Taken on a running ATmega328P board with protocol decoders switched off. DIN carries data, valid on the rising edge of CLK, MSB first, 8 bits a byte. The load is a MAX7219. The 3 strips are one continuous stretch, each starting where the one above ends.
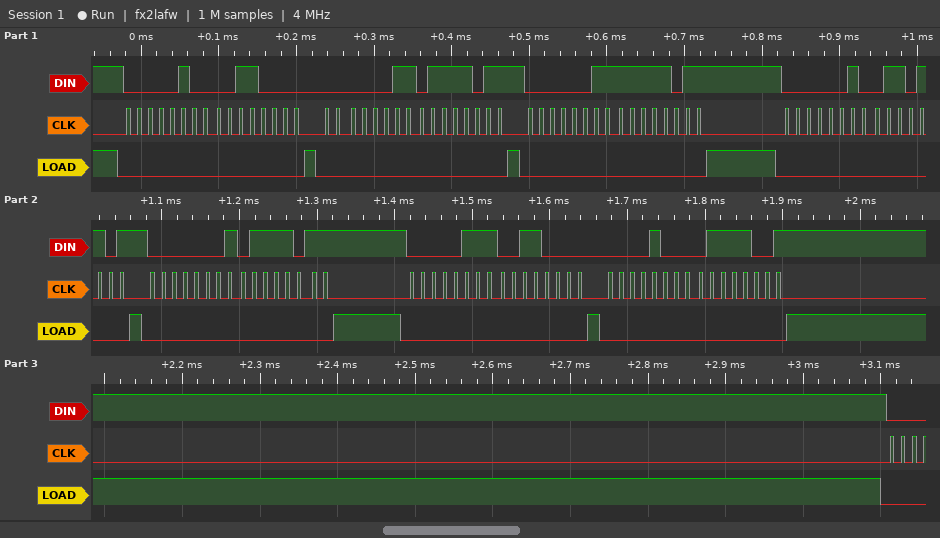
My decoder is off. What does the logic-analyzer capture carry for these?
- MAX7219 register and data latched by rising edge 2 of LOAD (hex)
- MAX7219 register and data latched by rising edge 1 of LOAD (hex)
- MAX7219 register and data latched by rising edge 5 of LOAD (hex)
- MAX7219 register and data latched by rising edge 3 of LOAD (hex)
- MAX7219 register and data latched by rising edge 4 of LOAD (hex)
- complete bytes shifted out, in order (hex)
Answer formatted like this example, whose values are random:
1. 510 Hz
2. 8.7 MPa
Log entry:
1. register 0x3, data 0x7B
2. register 0x4, data 0x30
3. register 0x1, data 0x7B
4. register 0x3, data 0xFB
5. register 0x2, data 0x6D
6. 04 30 03 7B 03 FB 02 6D 01 7B 07 30 08 79
